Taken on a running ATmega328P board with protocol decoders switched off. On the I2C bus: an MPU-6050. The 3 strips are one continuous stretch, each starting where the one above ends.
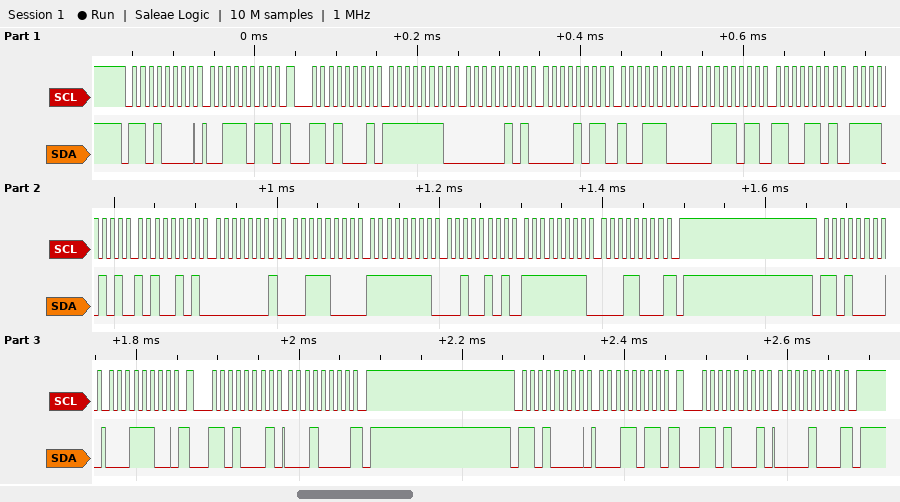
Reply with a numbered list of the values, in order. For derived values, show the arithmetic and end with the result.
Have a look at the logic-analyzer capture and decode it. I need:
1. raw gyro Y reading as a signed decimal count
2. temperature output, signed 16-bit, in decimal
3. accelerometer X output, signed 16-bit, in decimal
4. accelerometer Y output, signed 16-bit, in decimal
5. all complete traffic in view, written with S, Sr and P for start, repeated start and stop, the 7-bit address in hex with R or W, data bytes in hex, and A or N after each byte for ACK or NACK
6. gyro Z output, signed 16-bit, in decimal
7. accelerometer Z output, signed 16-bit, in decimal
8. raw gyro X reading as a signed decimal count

1. 0xFF25 = -219
2. 0xF5A5 = -2651
3. 0xFE05 = -507
4. 0x0B9C = 2972
5. S 68W A 3B A Sr 68R A FE A 05 A 0B A 9C A 3B A CD A F5 A A5 A 01 A 38 A FF A 25 A FF A 18 N P S 68W A 1C A Sr 68R A 10 N P S 68W A 1B A Sr 68R A 08 N P
6. 0xFF18 = -232
7. 0x3BCD = 15309
8. 0x0138 = 312
